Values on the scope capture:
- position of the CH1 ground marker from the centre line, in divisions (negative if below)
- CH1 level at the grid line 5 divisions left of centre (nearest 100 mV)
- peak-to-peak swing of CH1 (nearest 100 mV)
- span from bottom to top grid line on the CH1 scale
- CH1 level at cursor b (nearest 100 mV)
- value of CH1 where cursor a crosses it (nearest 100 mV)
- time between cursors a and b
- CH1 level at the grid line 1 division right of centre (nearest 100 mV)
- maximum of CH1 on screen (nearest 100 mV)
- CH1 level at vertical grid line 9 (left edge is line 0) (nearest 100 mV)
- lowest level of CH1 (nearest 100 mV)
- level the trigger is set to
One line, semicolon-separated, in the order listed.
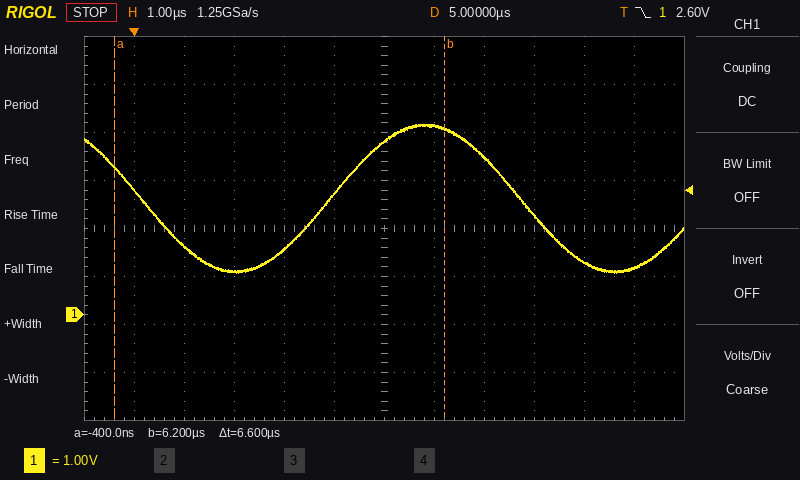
-1.8 div; 2.6 V; 3.1 V; 8 V; 3.9 V; 3.1 V; 6.6 µs; 3.9 V; 4.0 V; 2.1 V; 900 mV; 2.60 V
